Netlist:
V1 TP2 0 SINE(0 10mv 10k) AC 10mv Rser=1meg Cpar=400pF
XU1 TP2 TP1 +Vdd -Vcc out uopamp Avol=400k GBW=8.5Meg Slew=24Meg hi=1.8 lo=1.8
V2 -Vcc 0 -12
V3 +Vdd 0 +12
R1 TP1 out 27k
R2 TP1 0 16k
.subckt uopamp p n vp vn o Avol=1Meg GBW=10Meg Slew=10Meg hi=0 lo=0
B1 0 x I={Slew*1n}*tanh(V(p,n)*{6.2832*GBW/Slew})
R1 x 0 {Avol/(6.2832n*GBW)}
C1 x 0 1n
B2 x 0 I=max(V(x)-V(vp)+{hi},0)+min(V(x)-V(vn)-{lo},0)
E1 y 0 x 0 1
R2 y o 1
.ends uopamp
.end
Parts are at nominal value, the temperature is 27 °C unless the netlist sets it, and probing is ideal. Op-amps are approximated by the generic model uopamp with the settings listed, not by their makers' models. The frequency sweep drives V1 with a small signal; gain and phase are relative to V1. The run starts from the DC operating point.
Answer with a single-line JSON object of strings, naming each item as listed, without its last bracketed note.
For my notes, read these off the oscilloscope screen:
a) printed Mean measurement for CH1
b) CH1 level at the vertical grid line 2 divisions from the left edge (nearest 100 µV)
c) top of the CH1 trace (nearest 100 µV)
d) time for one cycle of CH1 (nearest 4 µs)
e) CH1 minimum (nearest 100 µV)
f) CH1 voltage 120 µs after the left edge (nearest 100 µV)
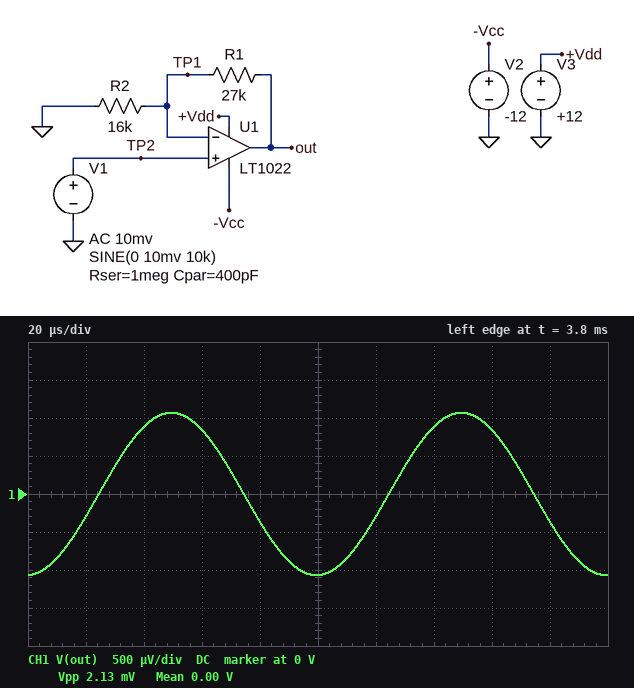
{"printed Mean measurement for CH1": "0.00 V", "CH1 level at the vertical grid line 2 divisions from the left edge": "900 µV", "top of the CH1 trace": "1.1 mV", "time for one cycle of CH1": "100 µs", "CH1 minimum": "-1.1 mV", "CH1 voltage 120 µs after the left edge": "-300 µV"}
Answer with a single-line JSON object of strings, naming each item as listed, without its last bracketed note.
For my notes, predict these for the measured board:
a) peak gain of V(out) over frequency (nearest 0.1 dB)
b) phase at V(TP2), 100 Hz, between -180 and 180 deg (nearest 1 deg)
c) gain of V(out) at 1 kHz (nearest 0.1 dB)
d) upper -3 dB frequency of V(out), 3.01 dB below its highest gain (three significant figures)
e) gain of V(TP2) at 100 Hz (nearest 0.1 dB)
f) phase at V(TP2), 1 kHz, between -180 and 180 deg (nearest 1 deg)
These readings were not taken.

{"peak gain of V(out) over frequency": "8.6 dB", "phase at V(TP2), 100 Hz, between -180 and 180 deg": "-14 deg", "gain of V(out) at 1 kHz": "-0.1 dB", "upper -3 dB frequency of V(out), 3.01 dB below its highest gain": "398 Hz", "gain of V(TP2) at 100 Hz": "-0.3 dB", "phase at V(TP2), 1 kHz, between -180 and 180 deg": "-68 deg"}
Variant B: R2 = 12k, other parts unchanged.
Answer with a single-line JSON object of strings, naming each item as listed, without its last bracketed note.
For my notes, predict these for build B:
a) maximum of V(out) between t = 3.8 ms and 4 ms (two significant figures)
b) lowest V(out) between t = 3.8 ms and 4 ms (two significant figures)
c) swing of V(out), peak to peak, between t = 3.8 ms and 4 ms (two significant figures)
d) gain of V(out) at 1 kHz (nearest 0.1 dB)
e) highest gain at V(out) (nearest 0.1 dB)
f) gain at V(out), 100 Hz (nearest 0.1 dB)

{"maximum of V(out) between t = 3.8 ms and 4 ms": "1.3 mV", "lowest V(out) between t = 3.8 ms and 4 ms": "-1.3 mV", "swing of V(out), peak to peak, between t = 3.8 ms and 4 ms": "2.6 mV", "gain of V(out) at 1 kHz": "1.6 dB", "highest gain at V(out)": "10.2 dB", "gain at V(out), 100 Hz": "10.0 dB"}
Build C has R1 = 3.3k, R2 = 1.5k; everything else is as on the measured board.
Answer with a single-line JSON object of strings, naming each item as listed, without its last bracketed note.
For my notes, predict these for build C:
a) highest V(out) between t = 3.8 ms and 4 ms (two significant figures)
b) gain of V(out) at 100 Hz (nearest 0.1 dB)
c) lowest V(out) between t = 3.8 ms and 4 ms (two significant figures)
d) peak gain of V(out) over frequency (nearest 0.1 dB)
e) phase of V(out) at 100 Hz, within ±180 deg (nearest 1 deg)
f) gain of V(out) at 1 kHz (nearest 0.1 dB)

{"highest V(out) between t = 3.8 ms and 4 ms": "1.3 mV", "gain of V(out) at 100 Hz": "9.8 dB", "lowest V(out) between t = 3.8 ms and 4 ms": "-1.3 mV", "peak gain of V(out) over frequency": "10.1 dB", "phase of V(out) at 100 Hz, within ±180 deg": "-14 deg", "gain of V(out) at 1 kHz": "1.5 dB"}
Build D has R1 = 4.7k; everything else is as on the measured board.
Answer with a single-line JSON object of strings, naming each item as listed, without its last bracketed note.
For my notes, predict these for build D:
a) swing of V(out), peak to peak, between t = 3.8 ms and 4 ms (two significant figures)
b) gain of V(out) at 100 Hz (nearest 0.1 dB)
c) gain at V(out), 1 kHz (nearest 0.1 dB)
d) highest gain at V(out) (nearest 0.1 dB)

{"swing of V(out), peak to peak, between t = 3.8 ms and 4 ms": "1.0 mV", "gain of V(out) at 100 Hz": "2.0 dB", "gain at V(out), 1 kHz": "-6.4 dB", "highest gain at V(out)": "2.2 dB"}
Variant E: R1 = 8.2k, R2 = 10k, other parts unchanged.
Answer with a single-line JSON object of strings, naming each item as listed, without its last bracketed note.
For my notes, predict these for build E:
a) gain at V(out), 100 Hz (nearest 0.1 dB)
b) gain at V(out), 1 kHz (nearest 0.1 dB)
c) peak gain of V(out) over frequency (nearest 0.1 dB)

{"gain at V(out), 100 Hz": "4.9 dB", "gain at V(out), 1 kHz": "-3.4 dB", "peak gain of V(out) over frequency": "5.2 dB"}
